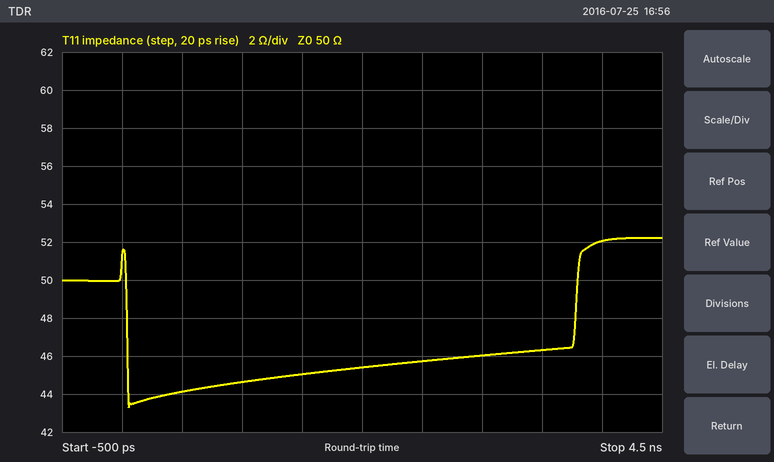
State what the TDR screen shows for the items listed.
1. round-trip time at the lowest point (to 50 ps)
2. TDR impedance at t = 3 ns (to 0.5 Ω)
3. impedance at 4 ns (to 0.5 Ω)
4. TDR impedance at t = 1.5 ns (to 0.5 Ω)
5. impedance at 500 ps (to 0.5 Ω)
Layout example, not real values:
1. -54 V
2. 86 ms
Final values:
1. 50 ps
2. 46.0 Ω
3. 52.0 Ω
4. 45.0 Ω
5. 44.0 Ω
